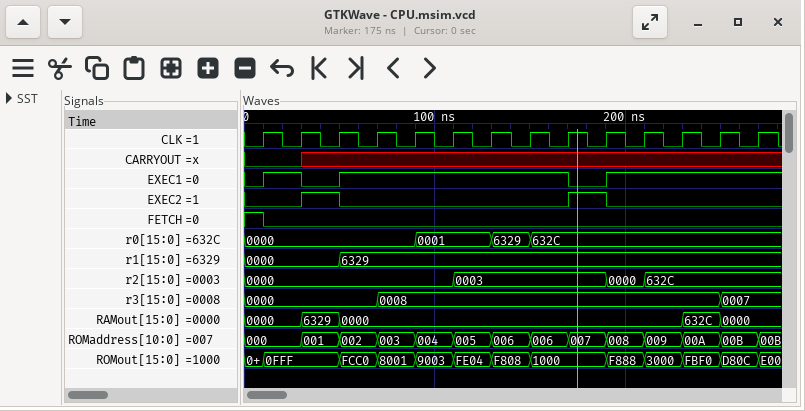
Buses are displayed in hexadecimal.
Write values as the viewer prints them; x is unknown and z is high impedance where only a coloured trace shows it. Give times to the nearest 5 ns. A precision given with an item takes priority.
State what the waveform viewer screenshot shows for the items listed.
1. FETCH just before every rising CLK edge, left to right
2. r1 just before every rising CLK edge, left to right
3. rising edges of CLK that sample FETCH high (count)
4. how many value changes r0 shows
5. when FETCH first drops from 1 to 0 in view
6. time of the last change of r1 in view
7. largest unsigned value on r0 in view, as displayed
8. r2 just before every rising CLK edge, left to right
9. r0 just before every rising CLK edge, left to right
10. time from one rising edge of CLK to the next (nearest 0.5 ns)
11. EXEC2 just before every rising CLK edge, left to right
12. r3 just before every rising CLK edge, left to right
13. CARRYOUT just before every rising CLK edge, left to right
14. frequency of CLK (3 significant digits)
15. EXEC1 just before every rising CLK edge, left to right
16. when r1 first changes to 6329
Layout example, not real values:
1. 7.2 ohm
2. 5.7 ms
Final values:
1. 1 0 0 0 0 0 0 0 0 0 0 0 0 0
2. 0000, 0000, 0000, 6329, 6329, 6329, 6329, 6329, 6329, 6329, 6329, 6329, 6329, 6329
3. 1
4. 3
5. 10 ns
6. 50 ns
7. 632C
8. 0000, 0000, 0000, 0000, 0000, 0000, 0003, 0003, 0003, 0003, 0000, 632C, 632C, 632C
9. 0000, 0000, 0000, 0000, 0000, 0001, 0001, 6329, 632C, 632C, 632C, 632C, 632C, 632C
10. 20 ns
11. 0 0 1 0 0 0 0 0 0 1 0 0 0 0
12. 0000, 0000, 0000, 0000, 0008, 0008, 0008, 0008, 0008, 0008, 0008, 0008, 0008, 0007
13. 0 0 x x x x x x x x x x x x
14. 50.0 MHz
15. 0 1 0 1 1 1 1 1 1 0 1 1 1 1
16. 50 ns
